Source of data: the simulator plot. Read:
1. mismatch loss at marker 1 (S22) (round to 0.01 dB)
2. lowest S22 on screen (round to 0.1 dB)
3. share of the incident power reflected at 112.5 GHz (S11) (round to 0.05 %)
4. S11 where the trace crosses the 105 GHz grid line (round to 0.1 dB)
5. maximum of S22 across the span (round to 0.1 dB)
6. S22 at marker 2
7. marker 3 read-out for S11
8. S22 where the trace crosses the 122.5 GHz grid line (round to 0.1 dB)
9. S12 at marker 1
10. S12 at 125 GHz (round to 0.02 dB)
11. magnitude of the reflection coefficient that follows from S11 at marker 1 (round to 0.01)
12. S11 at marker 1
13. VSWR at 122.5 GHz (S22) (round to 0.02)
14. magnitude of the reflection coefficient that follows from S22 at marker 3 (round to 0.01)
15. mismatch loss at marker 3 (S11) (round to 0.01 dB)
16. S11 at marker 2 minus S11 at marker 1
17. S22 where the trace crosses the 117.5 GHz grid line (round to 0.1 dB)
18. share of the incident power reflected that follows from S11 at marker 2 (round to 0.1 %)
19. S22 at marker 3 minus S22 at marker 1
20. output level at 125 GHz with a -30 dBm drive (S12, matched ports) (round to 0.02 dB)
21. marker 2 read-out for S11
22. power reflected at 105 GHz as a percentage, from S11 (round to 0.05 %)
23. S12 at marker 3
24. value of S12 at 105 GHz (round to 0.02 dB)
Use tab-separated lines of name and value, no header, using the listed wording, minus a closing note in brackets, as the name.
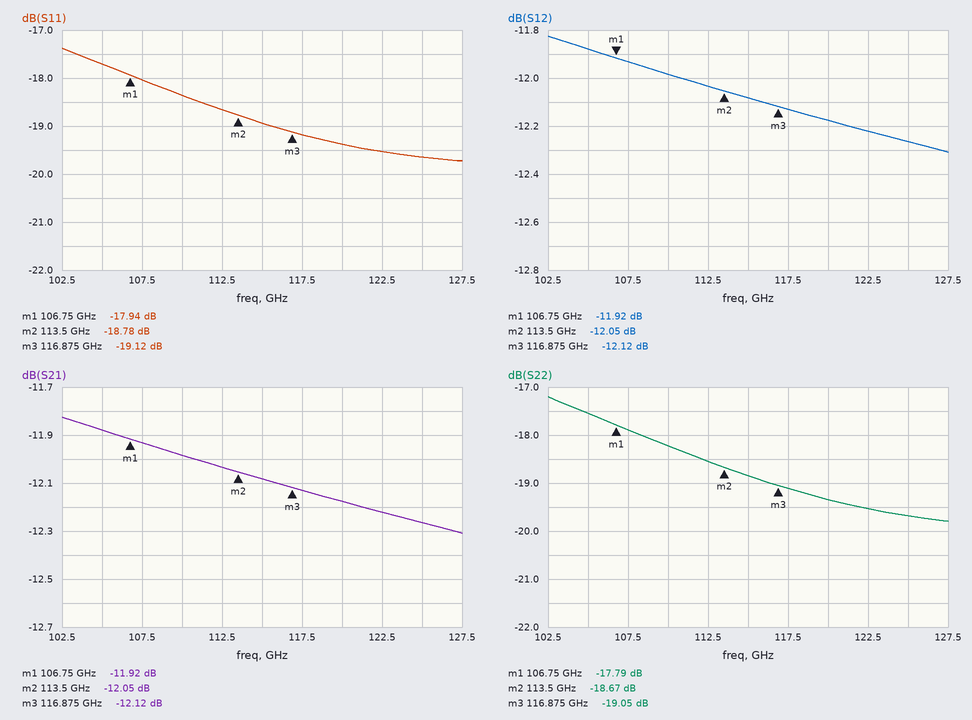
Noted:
mismatch loss at marker 1 (S22)	0.07 dB
lowest S22 on screen	-19.8 dB
share of the incident power reflected at 112.5 GHz (S11)	1.35 %
S11 where the trace crosses the 105 GHz grid line	-17.7 dB
maximum of S22 across the span	-17.2 dB
S22 at marker 2	-18.67 dB
marker 3 read-out for S11	-19.12 dB
S22 where the trace crosses the 122.5 GHz grid line	-19.5 dB
S12 at marker 1	-11.92 dB
S12 at 125 GHz	-12.26 dB
magnitude of the reflection coefficient that follows from S11 at marker 1	0.13
S11 at marker 1	-17.94 dB
VSWR at 122.5 GHz (S22)	1.24
magnitude of the reflection coefficient that follows from S22 at marker 3	0.11
mismatch loss at marker 3 (S11)	0.05 dB
S11 at marker 2 minus S11 at marker 1	-0.84 dB
S22 where the trace crosses the 117.5 GHz grid line	-19.1 dB
share of the incident power reflected that follows from S11 at marker 2	1.3 %
S22 at marker 3 minus S22 at marker 1	-1.26 dB
output level at 125 GHz with a -30 dBm drive (S12, matched ports)	-42.26 dBm
marker 2 read-out for S11	-18.78 dB
power reflected at 105 GHz as a percentage, from S11	1.70 %
S12 at marker 3	-12.12 dB
value of S12 at 105 GHz	-11.88 dB
